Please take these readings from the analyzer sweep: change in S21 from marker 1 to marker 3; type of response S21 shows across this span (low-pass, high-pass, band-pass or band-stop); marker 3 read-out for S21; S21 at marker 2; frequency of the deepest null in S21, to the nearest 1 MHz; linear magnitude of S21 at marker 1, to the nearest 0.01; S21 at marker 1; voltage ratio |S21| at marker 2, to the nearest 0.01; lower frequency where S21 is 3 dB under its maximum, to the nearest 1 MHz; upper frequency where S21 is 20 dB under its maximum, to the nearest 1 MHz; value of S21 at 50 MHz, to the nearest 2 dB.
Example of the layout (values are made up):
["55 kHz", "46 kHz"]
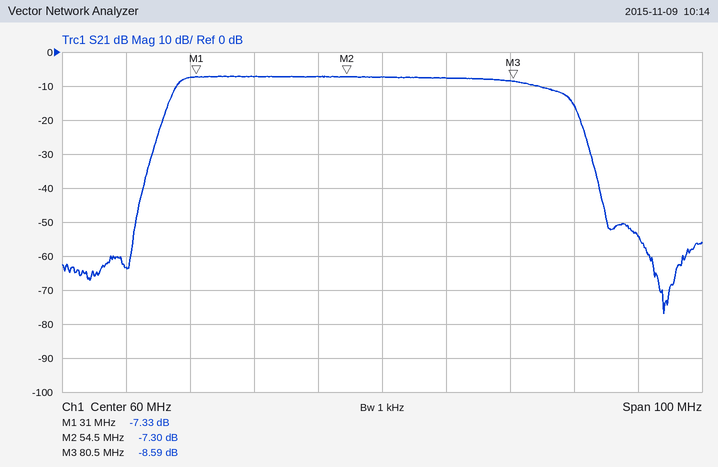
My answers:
["-1.26 dB", "band-pass", "-8.59 dB", "-7.30 dB", "104 MHz", "0.43", "-7.33 dB", "0.43", "28 MHz", "92 MHz", "-8 dB"]
